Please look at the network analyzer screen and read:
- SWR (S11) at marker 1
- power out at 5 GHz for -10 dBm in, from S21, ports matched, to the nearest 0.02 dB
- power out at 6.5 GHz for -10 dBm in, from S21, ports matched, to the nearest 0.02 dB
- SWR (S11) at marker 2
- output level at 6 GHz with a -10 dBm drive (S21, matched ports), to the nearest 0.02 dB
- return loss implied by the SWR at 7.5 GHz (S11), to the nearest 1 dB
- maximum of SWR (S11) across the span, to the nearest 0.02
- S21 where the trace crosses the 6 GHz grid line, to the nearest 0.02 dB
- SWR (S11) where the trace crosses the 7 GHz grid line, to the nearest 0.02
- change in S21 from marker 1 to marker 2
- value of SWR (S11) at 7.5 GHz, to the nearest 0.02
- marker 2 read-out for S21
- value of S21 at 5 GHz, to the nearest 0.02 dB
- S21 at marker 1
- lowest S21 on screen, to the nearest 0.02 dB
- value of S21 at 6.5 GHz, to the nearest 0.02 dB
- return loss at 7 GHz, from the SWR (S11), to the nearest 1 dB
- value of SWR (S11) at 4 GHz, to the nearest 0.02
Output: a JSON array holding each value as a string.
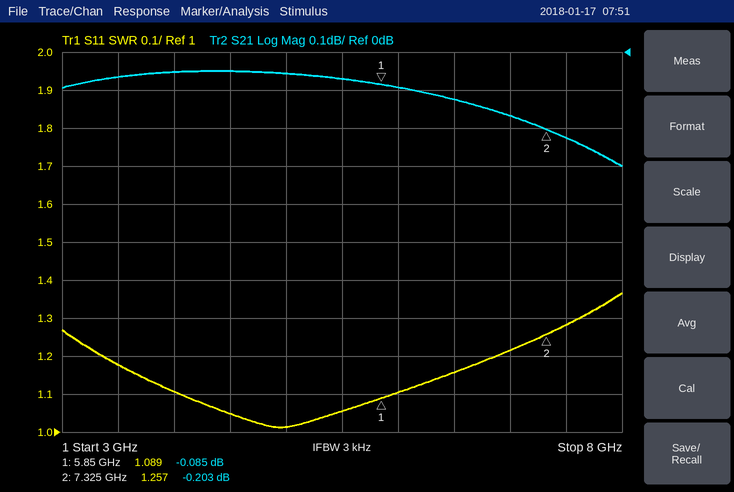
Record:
["1.089", "-10.06 dBm", "-10.12 dBm", "1.257", "-10.10 dBm", "18 dB", "1.36", "-0.10 dB", "1.22", "-0.118 dB", "1.28", "-0.203 dB", "-0.06 dB", "-0.085 dB", "-0.30 dB", "-0.12 dB", "20 dB", "1.10"]
